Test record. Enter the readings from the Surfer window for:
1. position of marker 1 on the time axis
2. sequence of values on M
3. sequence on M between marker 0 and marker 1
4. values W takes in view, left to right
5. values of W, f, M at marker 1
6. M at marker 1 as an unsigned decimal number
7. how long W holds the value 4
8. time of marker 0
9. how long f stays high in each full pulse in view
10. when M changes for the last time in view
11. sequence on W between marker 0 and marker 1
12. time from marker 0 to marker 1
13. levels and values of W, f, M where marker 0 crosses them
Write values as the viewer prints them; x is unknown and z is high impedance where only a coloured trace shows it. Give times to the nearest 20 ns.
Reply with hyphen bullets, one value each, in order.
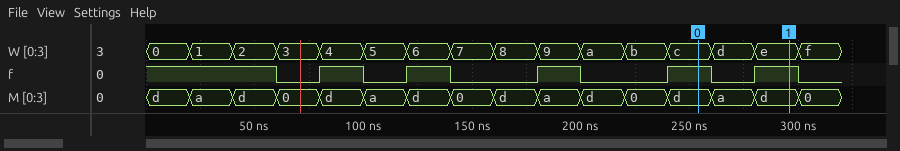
- 300 ns
- d, a, d, 0, d, a, d, 0, d, a, d, 0, d, a, d, 0
- d, a, d
- 0, 1, 2, 3, 4, 5, 6, 7, 8, 9, a, b, c, d, e, f
- W=e, f=1, M=d
- 13
- 20 ns
- 260 ns
- 20 ns, 20 ns, 20 ns, 20 ns, 20 ns
- 300 ns
- c, d, e
- 40 ns
- W=c, f=1, M=d
